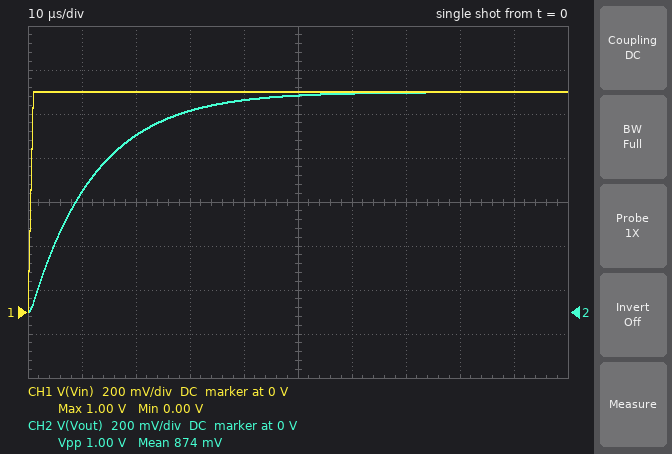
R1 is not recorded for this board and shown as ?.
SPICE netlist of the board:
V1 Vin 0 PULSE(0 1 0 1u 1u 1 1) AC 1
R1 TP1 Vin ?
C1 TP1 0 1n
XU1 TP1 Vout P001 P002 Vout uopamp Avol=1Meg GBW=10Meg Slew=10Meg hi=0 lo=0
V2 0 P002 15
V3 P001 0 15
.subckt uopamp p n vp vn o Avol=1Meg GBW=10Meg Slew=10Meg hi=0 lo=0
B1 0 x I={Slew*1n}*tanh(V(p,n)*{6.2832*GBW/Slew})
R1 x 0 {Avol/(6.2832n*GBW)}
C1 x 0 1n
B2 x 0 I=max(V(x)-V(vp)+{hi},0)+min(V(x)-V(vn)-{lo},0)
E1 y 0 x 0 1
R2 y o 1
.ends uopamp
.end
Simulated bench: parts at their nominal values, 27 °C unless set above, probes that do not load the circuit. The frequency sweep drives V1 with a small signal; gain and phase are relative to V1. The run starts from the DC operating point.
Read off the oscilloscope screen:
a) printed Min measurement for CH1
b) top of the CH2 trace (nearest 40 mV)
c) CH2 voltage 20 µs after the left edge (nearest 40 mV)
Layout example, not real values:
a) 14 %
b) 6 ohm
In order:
a) 0.00 V
b) 1.00 V
c) 800 mV
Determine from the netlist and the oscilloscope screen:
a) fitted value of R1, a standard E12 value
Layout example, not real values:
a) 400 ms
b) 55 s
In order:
a) 12 kΩ
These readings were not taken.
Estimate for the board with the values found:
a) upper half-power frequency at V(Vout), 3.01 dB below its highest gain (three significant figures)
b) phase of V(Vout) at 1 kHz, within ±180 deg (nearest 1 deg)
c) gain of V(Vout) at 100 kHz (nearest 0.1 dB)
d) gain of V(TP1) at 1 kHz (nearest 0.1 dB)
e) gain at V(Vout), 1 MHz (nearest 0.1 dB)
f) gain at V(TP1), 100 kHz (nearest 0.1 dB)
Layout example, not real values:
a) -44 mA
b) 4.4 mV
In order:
a) 13.3 kHz
b) -4 deg
c) -17.6 dB
d) 0 dB
e) -37.6 dB
f) -17.6 dB
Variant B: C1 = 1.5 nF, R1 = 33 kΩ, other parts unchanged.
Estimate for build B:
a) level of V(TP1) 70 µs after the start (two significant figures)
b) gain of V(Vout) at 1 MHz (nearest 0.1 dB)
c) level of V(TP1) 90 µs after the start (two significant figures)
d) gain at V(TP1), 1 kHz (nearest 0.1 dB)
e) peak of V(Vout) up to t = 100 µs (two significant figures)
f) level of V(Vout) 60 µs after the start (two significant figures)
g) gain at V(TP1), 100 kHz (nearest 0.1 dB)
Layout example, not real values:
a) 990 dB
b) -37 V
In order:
a) 750 mV
b) -49.9 dB
c) 840 mV
d) -0.4 dB
e) 870 mV
f) 700 mV
g) -29.9 dB
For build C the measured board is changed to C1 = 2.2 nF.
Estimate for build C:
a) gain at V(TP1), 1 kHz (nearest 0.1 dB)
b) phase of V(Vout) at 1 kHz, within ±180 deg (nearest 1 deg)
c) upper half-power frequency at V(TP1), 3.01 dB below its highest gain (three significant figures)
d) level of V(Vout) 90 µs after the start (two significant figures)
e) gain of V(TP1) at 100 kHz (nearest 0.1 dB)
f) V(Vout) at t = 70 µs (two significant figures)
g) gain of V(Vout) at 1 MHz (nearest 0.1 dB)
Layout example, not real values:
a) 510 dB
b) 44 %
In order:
a) -0.1 dB
b) -9 deg
c) 6.03 kHz
d) 970 mV
e) -24.4 dB
f) 930 mV
g) -44.4 dB
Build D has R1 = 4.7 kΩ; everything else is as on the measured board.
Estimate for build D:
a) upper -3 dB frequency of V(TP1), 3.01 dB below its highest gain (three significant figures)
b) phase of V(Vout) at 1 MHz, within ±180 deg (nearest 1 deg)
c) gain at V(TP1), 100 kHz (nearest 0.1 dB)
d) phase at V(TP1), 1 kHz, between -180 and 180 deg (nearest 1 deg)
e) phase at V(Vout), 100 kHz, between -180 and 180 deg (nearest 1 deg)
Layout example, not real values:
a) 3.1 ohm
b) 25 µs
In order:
a) 33.9 kHz
b) -94 deg
c) -9.9 dB
d) -2 deg
e) -72 deg
